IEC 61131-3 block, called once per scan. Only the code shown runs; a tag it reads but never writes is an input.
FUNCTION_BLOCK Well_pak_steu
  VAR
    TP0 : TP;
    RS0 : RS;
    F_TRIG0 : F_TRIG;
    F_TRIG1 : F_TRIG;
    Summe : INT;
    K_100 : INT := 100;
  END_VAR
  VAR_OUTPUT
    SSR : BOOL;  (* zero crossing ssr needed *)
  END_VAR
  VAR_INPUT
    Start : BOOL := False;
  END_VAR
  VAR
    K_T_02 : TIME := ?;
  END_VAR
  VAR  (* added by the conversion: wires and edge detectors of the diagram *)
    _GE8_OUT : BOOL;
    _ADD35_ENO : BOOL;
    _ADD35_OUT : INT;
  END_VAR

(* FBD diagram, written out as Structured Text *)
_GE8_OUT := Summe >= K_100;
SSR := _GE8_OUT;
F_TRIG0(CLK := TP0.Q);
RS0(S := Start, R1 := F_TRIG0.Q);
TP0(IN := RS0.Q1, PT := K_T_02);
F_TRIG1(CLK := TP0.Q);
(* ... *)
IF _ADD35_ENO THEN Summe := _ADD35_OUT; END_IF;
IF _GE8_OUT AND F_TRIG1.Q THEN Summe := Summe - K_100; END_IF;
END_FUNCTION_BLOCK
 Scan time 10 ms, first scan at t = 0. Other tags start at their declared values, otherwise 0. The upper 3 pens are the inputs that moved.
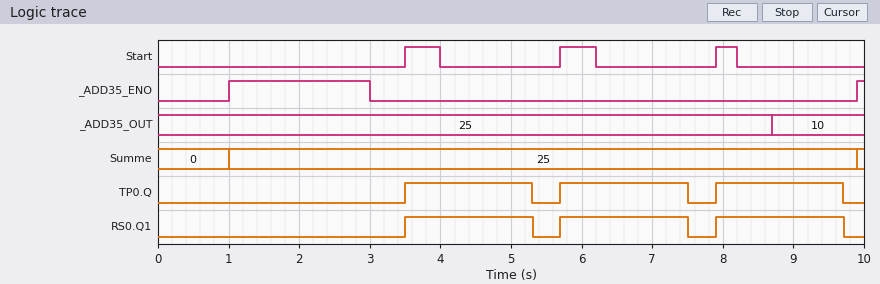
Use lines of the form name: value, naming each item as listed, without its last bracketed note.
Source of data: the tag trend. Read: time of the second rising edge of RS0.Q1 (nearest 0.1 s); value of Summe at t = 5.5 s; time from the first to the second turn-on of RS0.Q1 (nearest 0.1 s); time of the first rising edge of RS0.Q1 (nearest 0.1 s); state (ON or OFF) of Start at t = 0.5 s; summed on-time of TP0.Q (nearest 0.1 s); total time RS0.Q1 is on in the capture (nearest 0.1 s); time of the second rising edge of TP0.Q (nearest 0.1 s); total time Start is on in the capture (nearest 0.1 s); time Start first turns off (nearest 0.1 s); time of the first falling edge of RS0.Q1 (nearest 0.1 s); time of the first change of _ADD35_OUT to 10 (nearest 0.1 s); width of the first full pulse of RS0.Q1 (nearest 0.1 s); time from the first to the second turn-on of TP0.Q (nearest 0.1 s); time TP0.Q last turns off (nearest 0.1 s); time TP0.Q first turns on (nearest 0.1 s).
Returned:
time of the second rising edge of RS0.Q1: 5.7 s
value of Summe at t = 5.5 s: 25
time from the first to the second turn-on of RS0.Q1: 2.2 s
time of the first rising edge of RS0.Q1: 3.5 s
state (ON or OFF) of Start at t = 0.5 s: OFF
summed on-time of TP0.Q: 5.4 s
total time RS0.Q1 is on in the capture: 5.4 s
time of the second rising edge of TP0.Q: 5.7 s
total time Start is on in the capture: 1.3 s
time Start first turns off: 4.0 s
time of the first falling edge of RS0.Q1: 5.3 s
time of the first change of _ADD35_OUT to 10: 8.7 s
width of the first full pulse of RS0.Q1: 1.8 s
time from the first to the second turn-on of TP0.Q: 2.2 s
time TP0.Q last turns off: 9.7 s
time TP0.Q first turns on: 3.5 s
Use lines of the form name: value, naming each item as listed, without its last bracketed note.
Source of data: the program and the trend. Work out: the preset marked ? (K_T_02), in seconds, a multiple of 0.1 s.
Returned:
the preset marked ? (K_T_02), in seconds, a multiple of 0.1 s: 1.8 s
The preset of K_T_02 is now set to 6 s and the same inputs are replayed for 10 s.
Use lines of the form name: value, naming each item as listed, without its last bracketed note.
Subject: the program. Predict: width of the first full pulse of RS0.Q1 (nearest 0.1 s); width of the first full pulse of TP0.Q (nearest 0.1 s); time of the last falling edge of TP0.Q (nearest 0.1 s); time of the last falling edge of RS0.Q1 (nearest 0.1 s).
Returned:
width of the first full pulse of RS0.Q1: 6.0 s
width of the first full pulse of TP0.Q: 6.0 s
time of the last falling edge of TP0.Q: 9.5 s
time of the last falling edge of RS0.Q1: 9.5 s
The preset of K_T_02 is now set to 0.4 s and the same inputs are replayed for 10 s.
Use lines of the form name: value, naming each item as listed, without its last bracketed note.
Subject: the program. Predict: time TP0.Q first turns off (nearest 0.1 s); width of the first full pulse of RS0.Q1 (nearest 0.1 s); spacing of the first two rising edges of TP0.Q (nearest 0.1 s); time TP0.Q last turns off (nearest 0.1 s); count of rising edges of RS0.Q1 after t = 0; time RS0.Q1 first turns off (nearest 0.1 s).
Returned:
time TP0.Q first turns off: 3.9 s
width of the first full pulse of RS0.Q1: 0.4 s
spacing of the first two rising edges of TP0.Q: 0.4 s
time TP0.Q last turns off: 8.3 s
count of rising edges of RS0.Q1 after t = 0: 5
time RS0.Q1 first turns off: 3.9 s
